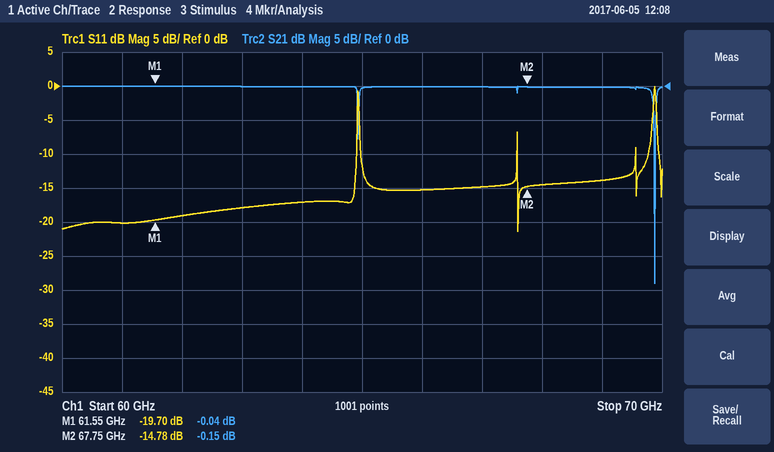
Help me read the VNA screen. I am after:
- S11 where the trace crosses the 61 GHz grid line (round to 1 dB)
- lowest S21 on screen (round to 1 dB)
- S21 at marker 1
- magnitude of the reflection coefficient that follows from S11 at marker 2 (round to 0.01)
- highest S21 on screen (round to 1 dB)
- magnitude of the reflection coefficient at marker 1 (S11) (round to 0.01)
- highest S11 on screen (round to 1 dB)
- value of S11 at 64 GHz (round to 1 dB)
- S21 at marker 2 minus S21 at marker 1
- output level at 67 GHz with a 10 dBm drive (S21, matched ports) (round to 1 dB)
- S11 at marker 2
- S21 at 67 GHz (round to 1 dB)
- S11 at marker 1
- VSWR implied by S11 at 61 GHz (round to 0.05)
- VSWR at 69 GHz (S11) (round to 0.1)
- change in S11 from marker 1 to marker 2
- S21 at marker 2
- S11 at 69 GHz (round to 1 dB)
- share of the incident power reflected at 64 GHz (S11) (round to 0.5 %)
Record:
-20 dB
-29 dB
-0.04 dB
0.18
0 dB
0.10
0 dB
-17 dB
-0.11 dB
10 dBm
-14.78 dB
0 dB
-19.70 dB
1.20
1.5
4.92 dB
-0.15 dB
-14 dB
2.0 %
